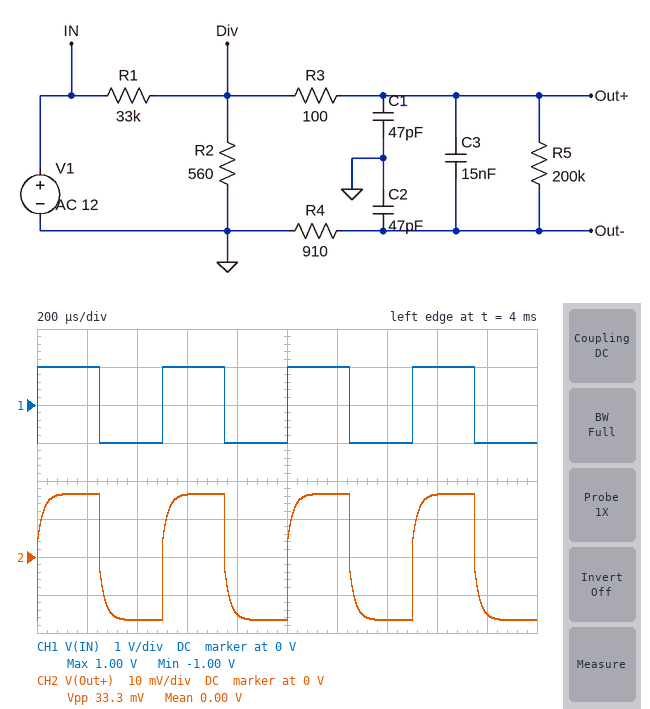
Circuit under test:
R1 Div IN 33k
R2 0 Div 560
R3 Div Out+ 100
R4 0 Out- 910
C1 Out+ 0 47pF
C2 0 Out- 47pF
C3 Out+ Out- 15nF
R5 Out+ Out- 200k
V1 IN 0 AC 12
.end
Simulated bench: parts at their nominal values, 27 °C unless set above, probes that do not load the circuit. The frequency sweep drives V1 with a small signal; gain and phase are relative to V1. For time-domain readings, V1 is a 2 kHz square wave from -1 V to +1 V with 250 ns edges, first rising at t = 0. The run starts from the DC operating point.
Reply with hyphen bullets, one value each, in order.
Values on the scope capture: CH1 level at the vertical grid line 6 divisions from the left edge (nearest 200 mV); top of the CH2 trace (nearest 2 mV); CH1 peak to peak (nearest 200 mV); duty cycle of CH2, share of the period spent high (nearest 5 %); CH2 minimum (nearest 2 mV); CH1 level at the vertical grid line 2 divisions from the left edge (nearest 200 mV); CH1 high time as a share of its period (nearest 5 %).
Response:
- 1.0 V
- 16 mV
- 2.0 V
- 50 %
- -16 mV
- -1.0 V
- 50 %
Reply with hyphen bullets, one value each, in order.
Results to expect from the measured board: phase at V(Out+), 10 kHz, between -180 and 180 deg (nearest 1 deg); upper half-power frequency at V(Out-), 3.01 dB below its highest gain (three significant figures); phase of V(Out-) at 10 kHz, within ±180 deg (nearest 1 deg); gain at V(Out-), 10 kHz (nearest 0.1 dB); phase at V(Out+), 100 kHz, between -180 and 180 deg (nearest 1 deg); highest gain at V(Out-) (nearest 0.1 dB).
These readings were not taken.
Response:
- -15 deg
- 4.48 MHz
- 34 deg
- -41.9 dB
- -4 deg
- -40.3 dB
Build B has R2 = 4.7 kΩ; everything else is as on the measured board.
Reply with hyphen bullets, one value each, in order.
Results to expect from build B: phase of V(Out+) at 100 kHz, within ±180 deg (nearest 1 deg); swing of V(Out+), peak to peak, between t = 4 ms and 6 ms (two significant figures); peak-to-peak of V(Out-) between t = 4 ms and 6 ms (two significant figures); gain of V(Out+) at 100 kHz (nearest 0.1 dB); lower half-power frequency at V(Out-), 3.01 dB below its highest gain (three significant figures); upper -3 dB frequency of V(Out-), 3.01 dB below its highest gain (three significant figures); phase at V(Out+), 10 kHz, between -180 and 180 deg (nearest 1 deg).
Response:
- -8 deg
- 230 mV
- 84 mV
- -33.0 dB
- 2.11 kHz
- 2.27 MHz
- -38 deg
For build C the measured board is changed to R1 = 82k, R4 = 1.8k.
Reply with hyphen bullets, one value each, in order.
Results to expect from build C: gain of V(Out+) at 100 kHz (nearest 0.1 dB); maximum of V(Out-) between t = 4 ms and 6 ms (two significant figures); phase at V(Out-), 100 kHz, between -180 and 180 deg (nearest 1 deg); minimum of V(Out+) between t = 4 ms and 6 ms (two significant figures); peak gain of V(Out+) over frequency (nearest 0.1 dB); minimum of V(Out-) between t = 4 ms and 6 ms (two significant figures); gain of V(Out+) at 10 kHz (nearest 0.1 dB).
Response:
- -46.1 dB
- 9.8 mV
- 1 deg
- -6.8 mV
- -43.4 dB
- -9.8 mV
- -45.5 dB
